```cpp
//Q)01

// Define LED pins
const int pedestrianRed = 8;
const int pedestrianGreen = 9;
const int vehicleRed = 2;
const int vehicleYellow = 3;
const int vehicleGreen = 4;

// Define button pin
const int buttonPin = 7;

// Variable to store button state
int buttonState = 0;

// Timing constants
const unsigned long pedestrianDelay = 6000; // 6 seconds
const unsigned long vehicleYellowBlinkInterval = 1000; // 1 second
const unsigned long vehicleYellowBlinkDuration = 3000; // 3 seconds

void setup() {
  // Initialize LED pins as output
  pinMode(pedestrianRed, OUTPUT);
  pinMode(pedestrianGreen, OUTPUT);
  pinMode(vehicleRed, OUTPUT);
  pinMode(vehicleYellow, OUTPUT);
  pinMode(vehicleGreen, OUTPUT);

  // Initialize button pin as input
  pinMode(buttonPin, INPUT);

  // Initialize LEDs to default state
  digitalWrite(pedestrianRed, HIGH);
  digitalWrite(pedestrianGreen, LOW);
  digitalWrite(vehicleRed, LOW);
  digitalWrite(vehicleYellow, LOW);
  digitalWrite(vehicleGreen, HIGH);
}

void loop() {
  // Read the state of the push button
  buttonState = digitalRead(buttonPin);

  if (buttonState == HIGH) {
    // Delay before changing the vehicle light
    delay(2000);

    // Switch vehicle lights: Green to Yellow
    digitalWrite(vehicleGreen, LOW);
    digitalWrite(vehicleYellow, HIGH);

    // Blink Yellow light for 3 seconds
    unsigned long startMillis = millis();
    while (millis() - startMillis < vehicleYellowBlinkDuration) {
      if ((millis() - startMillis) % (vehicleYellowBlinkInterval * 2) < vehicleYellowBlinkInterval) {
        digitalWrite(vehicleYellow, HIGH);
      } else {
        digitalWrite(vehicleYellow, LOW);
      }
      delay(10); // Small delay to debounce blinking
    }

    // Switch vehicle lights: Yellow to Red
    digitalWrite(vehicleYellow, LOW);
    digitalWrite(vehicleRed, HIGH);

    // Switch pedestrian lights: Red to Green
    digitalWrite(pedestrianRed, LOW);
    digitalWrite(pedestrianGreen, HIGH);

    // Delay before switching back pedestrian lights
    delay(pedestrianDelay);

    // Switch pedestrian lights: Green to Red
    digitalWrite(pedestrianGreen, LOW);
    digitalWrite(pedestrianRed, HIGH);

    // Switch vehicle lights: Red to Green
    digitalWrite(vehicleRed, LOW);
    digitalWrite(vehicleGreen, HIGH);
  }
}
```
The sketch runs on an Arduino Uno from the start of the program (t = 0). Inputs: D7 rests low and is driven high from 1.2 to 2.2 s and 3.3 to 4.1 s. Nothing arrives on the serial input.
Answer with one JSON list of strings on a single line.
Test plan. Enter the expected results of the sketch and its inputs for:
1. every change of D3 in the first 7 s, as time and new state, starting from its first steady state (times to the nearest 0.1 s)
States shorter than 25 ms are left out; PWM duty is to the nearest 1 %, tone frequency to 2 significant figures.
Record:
["0 s low; 3.2 s high; 4.2 s low; 5.2 s high; 6.2 s low"]
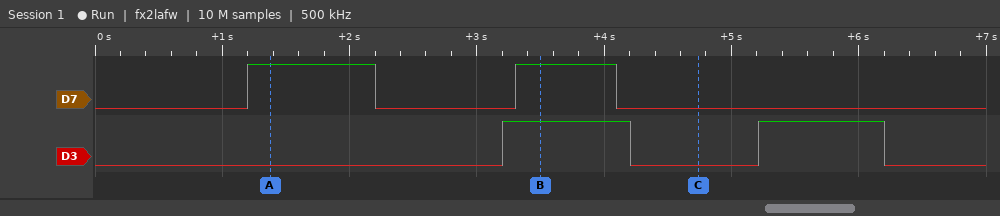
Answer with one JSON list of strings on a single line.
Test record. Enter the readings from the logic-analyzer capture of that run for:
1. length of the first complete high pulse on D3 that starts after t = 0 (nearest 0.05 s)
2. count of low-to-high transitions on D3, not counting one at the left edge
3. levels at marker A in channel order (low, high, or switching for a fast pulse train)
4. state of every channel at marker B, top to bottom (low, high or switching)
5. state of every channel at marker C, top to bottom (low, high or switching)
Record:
["1.00 s", "2", "D7 high, D3 low", "D7 high, D3 high", "D7 low, D3 low"]
